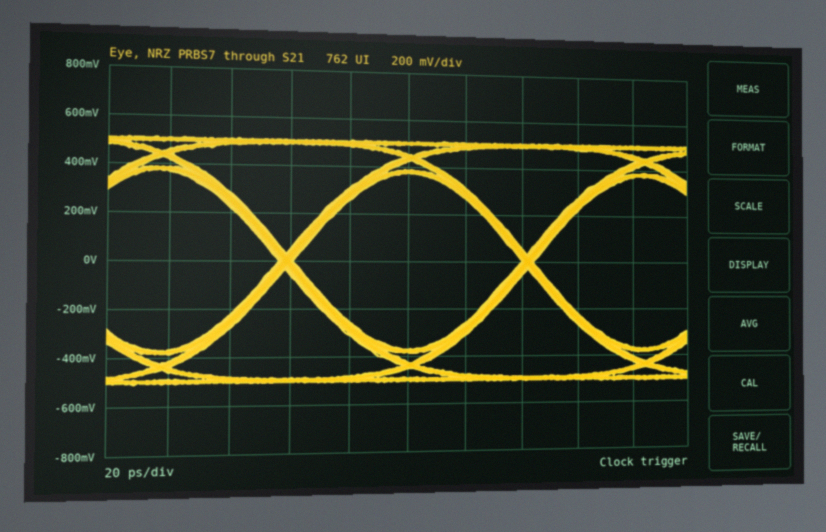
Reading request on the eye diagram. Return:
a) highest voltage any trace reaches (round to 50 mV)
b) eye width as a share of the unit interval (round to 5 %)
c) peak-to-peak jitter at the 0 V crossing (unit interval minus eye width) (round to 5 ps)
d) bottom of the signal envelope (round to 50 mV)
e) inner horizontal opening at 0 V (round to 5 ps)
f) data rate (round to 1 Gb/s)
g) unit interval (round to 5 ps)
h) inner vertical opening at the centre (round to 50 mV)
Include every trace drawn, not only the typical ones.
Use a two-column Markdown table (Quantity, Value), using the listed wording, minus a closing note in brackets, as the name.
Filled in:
| Quantity | Value |
|---|---|
| highest voltage any trace reaches | 500 mV |
| eye width as a share of the unit interval | 95 % |
| peak-to-peak jitter at the 0 V crossing (unit interval minus eye width) | 5 ps |
| bottom of the signal envelope | -500 mV |
| inner horizontal opening at 0 V | 80 ps |
| data rate | 12 Gb/s |
| unit interval | 85 ps |
| inner vertical opening at the centre | 750 mV |
